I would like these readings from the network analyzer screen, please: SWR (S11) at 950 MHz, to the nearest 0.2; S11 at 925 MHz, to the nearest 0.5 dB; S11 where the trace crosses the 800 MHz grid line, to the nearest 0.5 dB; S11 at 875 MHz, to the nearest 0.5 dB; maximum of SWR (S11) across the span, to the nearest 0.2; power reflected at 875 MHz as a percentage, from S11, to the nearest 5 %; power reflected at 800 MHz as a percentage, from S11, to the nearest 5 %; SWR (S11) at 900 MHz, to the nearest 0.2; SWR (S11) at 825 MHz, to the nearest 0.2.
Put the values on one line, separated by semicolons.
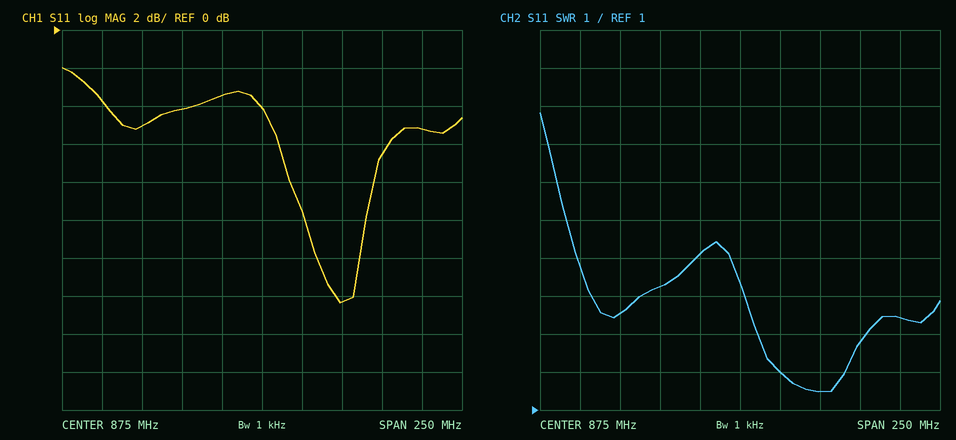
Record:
2.8; -14.5 dB; -5.0 dB; -4.0 dB; 8.8; 40 %; 30 %; 2.0; 4.2
